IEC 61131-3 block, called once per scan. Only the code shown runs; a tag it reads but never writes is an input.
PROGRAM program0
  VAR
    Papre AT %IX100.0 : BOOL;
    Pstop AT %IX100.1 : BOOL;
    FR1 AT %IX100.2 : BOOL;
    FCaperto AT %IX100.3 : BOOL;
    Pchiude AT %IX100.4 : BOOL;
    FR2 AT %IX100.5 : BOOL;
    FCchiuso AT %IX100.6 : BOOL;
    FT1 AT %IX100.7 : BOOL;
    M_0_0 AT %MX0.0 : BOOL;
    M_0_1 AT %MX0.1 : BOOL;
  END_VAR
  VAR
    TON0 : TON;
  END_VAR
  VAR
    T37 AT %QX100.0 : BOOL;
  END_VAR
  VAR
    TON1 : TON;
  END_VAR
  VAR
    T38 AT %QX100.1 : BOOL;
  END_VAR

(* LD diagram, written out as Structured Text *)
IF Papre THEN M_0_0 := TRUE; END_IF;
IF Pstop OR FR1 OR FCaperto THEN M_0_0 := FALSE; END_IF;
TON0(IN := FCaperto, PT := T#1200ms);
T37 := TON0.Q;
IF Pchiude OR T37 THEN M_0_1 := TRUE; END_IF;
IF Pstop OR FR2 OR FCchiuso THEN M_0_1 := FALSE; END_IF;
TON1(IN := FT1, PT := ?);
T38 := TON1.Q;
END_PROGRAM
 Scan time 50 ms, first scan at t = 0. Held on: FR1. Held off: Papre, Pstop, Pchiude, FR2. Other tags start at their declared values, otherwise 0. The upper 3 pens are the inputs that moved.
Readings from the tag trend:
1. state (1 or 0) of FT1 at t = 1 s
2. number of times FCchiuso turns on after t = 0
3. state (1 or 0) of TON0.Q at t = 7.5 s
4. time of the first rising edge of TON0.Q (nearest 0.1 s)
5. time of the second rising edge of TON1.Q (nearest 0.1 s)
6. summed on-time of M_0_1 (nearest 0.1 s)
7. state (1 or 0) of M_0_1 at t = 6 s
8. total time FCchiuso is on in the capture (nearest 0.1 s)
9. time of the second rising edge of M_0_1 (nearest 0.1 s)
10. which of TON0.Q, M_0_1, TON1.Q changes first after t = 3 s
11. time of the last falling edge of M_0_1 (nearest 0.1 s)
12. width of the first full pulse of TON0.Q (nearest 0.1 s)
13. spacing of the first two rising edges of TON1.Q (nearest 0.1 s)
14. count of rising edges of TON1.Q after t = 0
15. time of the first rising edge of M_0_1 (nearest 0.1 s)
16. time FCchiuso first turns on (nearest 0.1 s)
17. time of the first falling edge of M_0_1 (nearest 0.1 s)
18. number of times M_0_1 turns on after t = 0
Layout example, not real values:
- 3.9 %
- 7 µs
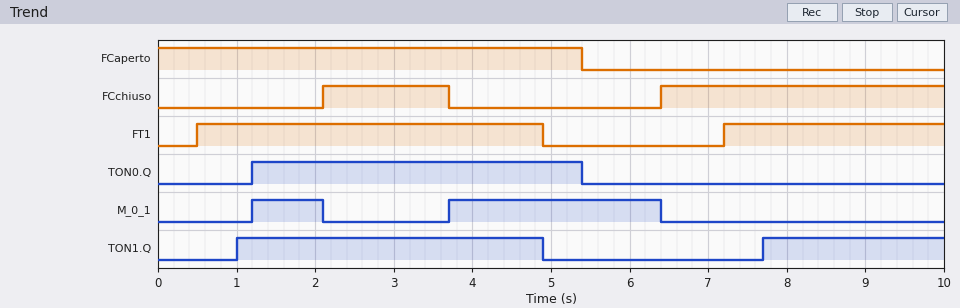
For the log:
- 1
- 2
- 0
- 1.2 s
- 7.7 s
- 3.6 s
- 1
- 5.2 s
- 3.7 s
- M_0_1
- 6.4 s
- 4.2 s
- 6.7 s
- 2
- 1.2 s
- 2.1 s
- 2.1 s
- 2
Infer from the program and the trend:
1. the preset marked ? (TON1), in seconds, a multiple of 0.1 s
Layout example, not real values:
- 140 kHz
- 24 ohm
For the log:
- 0.5 s
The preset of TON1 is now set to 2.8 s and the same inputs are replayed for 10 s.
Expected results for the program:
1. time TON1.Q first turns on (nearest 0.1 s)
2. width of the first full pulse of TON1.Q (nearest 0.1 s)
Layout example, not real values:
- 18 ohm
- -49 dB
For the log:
- 3.3 s
- 1.6 s
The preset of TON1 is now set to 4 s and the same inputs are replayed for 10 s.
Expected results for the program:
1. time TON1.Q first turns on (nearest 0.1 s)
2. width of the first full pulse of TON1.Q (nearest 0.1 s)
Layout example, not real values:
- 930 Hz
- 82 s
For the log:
- 4.5 s
- 0.4 s
